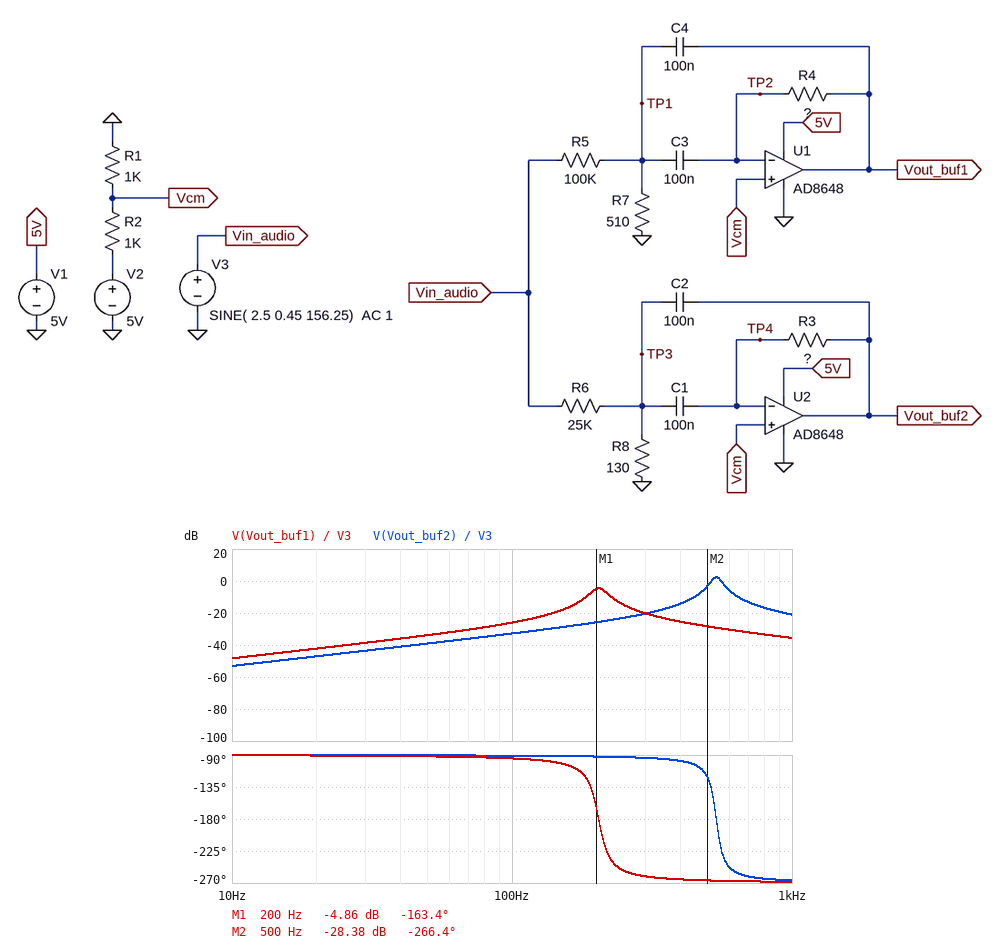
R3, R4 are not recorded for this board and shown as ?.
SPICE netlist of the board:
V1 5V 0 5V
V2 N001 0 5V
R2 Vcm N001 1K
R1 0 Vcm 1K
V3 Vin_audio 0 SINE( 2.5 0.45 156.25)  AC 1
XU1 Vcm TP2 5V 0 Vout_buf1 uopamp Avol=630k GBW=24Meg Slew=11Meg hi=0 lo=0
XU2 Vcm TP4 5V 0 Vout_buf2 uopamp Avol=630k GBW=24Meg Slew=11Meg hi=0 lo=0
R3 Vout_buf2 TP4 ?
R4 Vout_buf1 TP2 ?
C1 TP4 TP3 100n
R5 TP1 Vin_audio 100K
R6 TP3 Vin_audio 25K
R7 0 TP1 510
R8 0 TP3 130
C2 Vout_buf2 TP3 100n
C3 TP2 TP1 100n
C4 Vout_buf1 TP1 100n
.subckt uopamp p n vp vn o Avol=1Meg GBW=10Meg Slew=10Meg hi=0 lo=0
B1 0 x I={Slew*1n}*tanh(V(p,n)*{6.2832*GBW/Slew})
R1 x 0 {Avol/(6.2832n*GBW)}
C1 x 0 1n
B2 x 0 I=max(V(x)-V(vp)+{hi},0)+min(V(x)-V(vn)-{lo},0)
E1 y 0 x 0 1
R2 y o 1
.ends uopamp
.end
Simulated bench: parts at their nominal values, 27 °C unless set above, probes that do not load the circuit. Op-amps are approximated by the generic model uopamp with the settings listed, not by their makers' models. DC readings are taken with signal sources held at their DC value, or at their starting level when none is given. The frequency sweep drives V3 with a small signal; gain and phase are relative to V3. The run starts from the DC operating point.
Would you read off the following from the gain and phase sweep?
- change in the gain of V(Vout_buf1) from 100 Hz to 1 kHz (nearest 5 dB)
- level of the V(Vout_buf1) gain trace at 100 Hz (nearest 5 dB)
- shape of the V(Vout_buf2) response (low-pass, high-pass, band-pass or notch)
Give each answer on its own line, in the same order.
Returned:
-10 dB
-25 dB
band-pass
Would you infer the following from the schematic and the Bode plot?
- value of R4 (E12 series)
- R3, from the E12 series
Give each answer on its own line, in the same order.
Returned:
120 kΩ
68 kΩ
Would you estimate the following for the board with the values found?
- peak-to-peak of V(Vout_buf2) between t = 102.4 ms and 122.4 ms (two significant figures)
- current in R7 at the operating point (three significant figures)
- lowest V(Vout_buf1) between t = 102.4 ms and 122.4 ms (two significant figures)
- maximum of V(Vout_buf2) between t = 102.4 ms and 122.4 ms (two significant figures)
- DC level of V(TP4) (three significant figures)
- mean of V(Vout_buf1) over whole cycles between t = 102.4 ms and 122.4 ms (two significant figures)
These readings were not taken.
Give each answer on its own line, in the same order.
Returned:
34 mV
24.9 µA
2.4 V
2.5 V
2.50 V
2.5 V
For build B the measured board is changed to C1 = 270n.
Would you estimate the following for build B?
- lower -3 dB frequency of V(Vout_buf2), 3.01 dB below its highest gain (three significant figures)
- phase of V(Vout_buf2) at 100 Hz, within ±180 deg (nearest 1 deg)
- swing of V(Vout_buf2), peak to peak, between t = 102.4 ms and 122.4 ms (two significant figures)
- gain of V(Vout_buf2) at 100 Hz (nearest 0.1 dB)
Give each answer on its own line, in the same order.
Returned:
311 Hz
-92 deg
110 mV
-23.6 dB
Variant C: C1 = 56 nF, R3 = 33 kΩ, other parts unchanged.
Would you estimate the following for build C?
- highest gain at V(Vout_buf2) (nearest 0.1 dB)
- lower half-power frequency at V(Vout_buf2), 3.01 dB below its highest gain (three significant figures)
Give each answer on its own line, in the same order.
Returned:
-6.5 dB
964 Hz
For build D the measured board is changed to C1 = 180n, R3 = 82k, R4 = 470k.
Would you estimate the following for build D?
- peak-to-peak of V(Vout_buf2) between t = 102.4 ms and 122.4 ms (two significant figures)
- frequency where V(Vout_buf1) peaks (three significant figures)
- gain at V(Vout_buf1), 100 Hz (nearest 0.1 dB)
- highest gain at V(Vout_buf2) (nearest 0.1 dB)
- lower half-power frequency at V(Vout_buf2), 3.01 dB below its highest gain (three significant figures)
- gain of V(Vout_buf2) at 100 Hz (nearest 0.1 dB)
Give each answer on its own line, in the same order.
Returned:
83 mV
103 Hz
4.8 dB
6.5 dB
349 Hz
-25.7 dB
